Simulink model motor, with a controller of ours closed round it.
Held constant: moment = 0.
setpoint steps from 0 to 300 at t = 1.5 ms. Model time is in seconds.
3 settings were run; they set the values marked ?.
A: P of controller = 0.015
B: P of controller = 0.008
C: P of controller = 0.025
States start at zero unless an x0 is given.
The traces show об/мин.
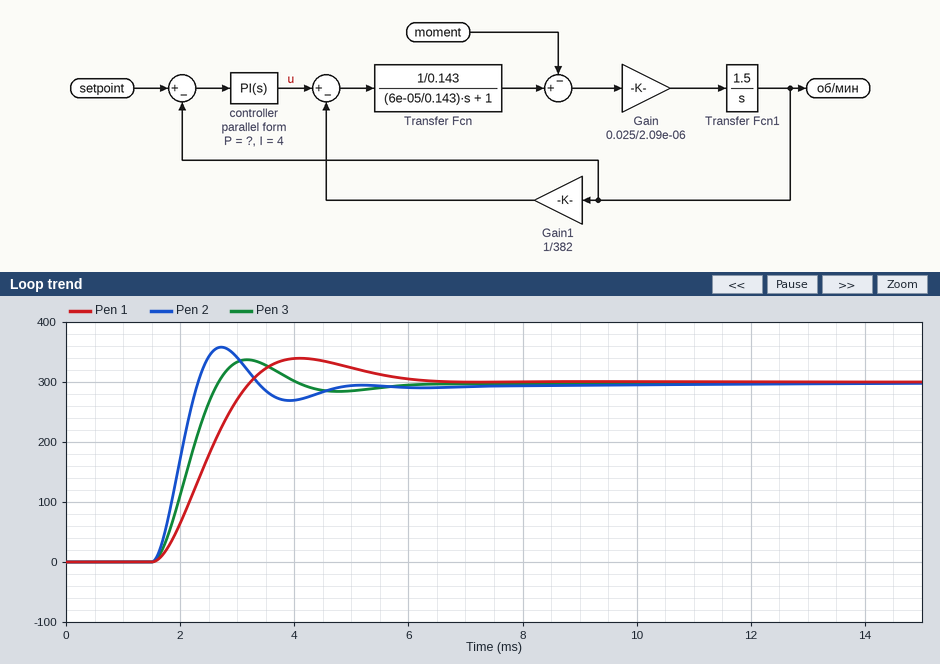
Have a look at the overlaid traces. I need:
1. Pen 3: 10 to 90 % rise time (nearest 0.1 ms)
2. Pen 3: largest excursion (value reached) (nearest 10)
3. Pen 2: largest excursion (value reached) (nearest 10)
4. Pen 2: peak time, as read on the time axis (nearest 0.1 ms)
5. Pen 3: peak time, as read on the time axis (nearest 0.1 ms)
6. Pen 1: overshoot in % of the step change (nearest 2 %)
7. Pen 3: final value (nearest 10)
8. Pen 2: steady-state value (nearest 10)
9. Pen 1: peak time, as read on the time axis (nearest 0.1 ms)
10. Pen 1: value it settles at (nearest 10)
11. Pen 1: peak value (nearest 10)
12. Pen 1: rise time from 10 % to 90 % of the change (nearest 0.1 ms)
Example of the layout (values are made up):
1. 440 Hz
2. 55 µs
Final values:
1. 0.8 ms
2. 340
3. 360
4. 2.7 ms
5. 3.2 ms
6. 14 %
7. 300
8. 300
9. 4.1 ms
10. 300
11. 340
12. 1.2 ms
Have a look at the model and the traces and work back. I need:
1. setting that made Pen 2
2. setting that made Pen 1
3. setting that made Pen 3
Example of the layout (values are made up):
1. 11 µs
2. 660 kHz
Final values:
1. C
2. B
3. A
